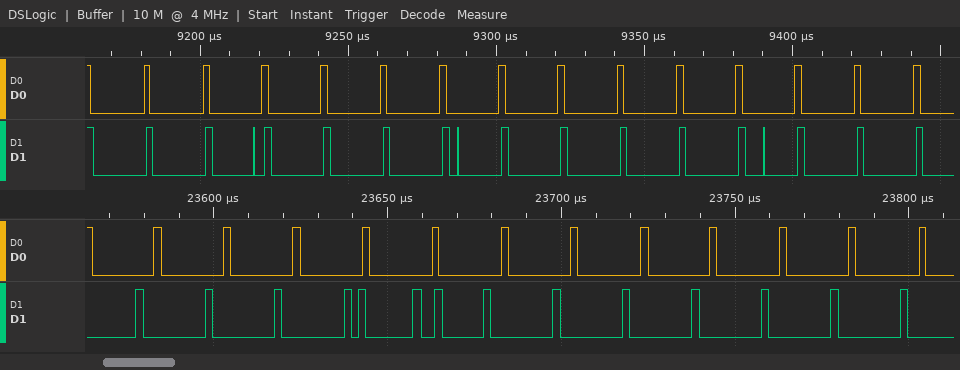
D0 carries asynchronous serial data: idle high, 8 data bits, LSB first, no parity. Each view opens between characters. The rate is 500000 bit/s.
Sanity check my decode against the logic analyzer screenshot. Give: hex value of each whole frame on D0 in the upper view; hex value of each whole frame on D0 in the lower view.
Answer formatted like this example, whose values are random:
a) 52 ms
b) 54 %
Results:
a) 00, 00, 00, 00, 00, 00, 00, 00, 00, 00, 00, 00, 00, 00
b) 00, 00, 00, 00, 00, 00, 00, 00, 00, 00, 00, 00
